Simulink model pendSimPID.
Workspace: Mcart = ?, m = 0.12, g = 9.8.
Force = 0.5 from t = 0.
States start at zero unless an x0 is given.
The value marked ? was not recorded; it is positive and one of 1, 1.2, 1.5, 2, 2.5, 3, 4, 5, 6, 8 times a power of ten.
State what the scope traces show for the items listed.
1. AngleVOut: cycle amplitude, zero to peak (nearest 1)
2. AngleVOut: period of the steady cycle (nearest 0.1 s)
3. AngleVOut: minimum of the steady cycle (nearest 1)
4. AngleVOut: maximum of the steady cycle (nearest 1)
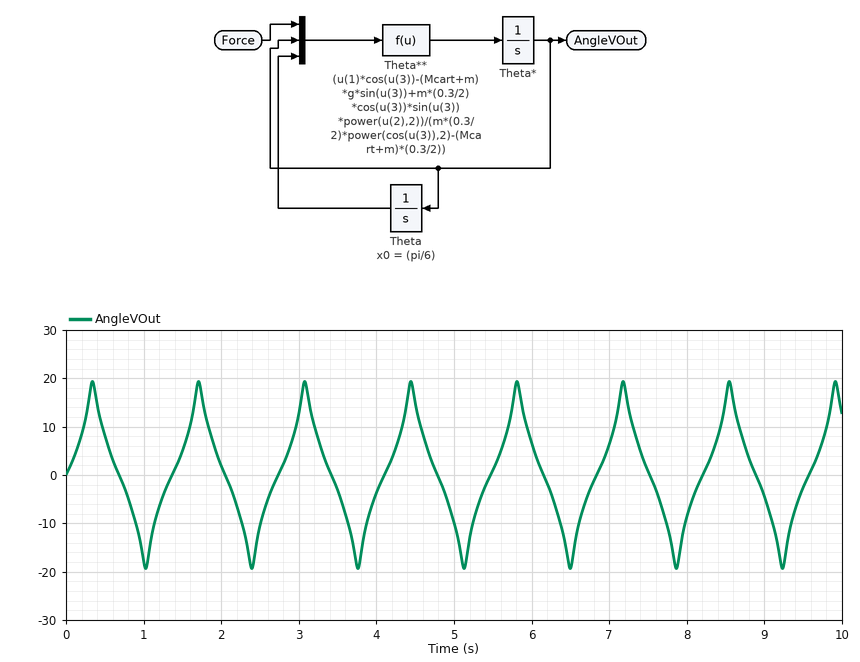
19
1.4 s
-19
19
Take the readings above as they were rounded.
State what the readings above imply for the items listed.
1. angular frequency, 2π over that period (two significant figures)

4.5 rad/s
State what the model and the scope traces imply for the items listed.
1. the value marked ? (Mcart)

0.25
